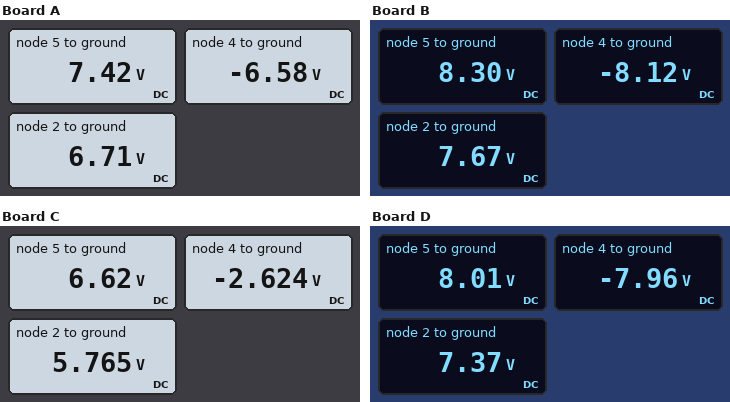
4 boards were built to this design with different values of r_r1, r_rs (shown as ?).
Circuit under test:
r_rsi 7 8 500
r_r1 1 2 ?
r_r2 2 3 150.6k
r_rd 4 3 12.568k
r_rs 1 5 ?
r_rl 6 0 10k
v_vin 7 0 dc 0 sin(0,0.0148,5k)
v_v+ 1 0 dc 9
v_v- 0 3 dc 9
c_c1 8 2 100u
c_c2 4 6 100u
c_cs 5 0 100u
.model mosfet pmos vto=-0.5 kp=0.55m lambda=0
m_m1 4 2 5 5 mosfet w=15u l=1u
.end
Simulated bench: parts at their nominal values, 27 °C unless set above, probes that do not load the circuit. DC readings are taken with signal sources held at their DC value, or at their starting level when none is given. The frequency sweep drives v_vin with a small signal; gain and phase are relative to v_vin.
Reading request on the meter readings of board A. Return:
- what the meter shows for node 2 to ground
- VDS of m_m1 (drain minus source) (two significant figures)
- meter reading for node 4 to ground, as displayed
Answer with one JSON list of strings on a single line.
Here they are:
["6.71 V", "-14 V", "-6.58 V"]
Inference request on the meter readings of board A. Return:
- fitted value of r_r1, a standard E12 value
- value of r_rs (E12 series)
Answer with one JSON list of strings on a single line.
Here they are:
["22 kΩ", "8.2 kΩ"]
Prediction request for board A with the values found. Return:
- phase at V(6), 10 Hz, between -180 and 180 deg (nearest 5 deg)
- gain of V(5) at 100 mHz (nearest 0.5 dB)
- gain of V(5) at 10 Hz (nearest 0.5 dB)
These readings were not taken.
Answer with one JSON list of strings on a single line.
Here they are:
["-165 deg", "-3.0 dB", "-11.5 dB"]
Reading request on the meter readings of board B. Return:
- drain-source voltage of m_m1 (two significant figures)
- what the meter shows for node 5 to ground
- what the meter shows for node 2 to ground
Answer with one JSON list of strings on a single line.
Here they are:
["-16 V", "8.30 V", "7.67 V"]
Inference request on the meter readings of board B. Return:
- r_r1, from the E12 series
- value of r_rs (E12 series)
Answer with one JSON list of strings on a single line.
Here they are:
["12 kΩ", "10 kΩ"]
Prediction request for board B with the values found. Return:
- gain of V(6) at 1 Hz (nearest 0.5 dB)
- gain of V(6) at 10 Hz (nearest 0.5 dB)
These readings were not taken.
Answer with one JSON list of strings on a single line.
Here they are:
["8.5 dB", "15.0 dB"]
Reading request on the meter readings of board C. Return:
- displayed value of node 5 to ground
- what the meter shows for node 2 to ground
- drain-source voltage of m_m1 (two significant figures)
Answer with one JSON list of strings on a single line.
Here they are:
["6.62 V", "5.765 V", "-9.2 V"]
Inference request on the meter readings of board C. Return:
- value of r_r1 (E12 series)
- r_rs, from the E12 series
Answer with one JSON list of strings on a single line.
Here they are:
["33 kΩ", "4.7 kΩ"]
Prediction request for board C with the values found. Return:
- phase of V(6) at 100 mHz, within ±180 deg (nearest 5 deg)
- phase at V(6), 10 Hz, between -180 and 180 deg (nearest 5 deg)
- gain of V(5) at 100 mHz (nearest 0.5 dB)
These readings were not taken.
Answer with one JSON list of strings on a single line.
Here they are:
["-100 deg", "-155 deg", "-2.0 dB"]
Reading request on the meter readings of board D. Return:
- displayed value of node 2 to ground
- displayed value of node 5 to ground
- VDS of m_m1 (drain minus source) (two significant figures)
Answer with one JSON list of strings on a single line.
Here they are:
["7.37 V", "8.01 V", "-16 V"]
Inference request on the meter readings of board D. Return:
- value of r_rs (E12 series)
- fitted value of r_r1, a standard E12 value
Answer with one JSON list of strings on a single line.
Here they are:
["12 kΩ", "15 kΩ"]
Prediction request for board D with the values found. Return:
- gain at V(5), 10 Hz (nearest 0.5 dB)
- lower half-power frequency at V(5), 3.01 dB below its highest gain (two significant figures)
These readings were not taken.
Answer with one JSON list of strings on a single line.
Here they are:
["-15.0 dB", "100 mHz"]
